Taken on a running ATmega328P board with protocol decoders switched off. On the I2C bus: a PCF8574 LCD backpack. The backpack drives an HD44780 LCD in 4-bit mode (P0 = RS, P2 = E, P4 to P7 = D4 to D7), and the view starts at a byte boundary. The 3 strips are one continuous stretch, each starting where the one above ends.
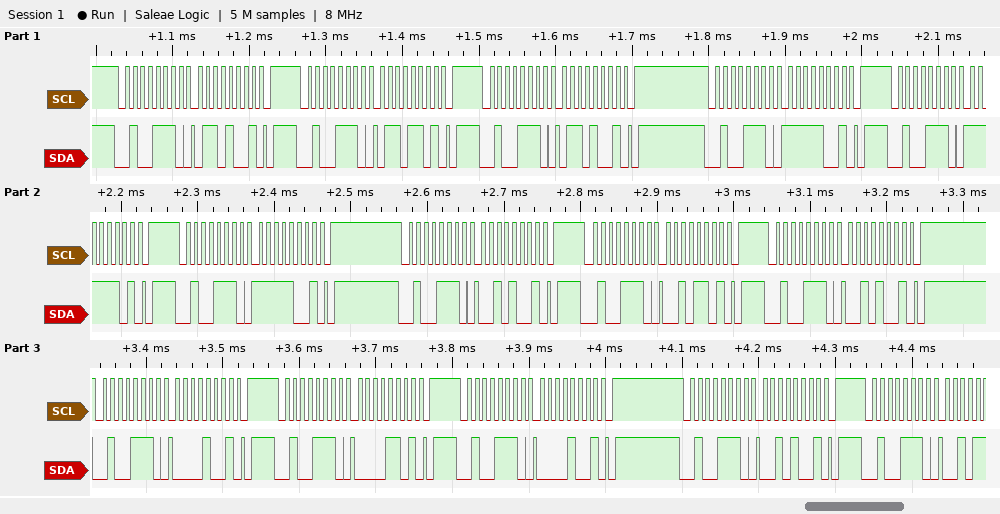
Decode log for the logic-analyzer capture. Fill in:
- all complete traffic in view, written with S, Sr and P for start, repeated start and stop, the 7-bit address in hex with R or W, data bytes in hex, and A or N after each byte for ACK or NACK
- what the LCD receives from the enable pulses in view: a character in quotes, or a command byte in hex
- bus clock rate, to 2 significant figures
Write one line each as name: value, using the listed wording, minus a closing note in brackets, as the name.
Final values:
all complete traffic in view, written with S, Sr and P for start, repeated start and stop, the 7-bit address in hex with R or W, data bytes in hex, and A or N after each byte for ACK or NACK: S 27W A 69 A P S 27W A 6D A P S 27W A 69 A P S 27W A F9 A P S 27W A FD A P S 27W A F9 A P S 27W A 29 A P S 27W A 2D A P S 27W A 29 A P S 27W A 09 A P S 27W A 0D A P S 27W A 09 A P S 27W A 29 A P S 27W A
what the LCD receives from the enable pulses in view: a character in quotes, or a command byte in hex: 'o' ' '
bus clock rate, to 2 significant figures: 100 kHz
